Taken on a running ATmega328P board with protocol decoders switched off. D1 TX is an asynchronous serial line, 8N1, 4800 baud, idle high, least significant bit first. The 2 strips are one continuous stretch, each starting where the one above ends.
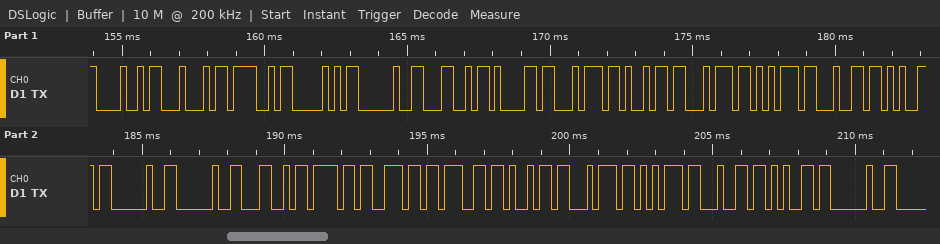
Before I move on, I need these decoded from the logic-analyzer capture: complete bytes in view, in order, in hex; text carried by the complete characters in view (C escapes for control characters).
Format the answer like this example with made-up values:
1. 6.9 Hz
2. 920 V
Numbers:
1. 0x48 0x44 0x4F 0x50 0x20 0x4C 0x61 0x74 0x69 0x74 0x75 0x64 0x65 0x20 0x20 0x4C 0x6F 0x6E 0x67 0x69 0x74 0x75 0x64 0x65 0x20
2. "HDOP Latitude  Longitude "
